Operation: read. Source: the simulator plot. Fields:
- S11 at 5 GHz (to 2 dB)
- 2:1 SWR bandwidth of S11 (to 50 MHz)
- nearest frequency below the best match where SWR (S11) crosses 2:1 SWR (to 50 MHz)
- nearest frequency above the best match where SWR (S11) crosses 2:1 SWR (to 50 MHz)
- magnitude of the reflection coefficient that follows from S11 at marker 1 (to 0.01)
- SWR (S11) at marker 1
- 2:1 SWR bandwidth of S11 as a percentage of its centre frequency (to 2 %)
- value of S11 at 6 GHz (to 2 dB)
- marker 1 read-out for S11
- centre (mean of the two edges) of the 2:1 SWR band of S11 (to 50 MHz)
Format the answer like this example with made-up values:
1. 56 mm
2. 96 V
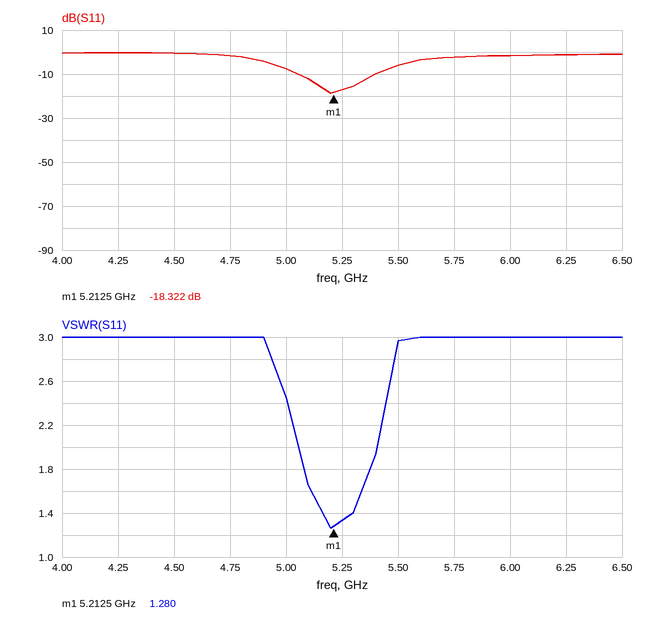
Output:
1. -8 dB
2. 350 MHz
3. 5.05 GHz
4. 5.40 GHz
5. 0.12
6. 1.280
7. 6 %
8. -2 dB
9. -18.322 dB
10. 5.25 GHz
